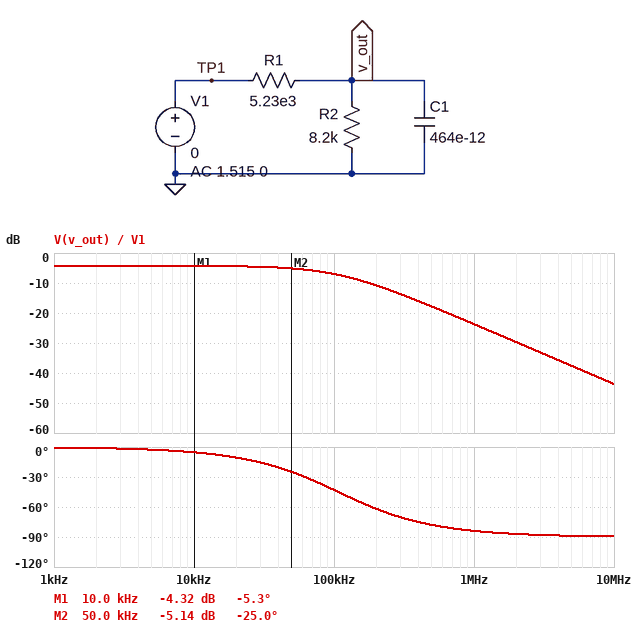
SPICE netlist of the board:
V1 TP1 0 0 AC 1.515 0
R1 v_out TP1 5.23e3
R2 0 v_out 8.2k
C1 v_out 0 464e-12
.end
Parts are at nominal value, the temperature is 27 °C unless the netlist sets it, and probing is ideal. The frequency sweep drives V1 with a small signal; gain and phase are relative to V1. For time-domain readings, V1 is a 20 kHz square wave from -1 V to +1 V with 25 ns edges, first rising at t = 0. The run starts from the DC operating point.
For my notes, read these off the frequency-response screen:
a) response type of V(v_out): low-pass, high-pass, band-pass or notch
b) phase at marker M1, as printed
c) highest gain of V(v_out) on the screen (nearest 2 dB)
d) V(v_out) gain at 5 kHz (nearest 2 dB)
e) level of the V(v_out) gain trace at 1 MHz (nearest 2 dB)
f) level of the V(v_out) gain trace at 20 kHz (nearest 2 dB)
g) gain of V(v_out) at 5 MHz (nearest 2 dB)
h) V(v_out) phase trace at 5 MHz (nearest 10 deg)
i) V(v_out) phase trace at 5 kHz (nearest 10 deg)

low-pass
-5.3 deg
-4 dB
-4 dB
-24 dB
-4 dB
-38 dB
-90 deg
0 deg
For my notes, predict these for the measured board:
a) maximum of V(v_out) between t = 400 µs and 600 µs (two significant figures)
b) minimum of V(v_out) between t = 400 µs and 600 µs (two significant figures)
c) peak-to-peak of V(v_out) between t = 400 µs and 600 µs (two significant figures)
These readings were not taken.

610 mV
-610 mV
1.2 V
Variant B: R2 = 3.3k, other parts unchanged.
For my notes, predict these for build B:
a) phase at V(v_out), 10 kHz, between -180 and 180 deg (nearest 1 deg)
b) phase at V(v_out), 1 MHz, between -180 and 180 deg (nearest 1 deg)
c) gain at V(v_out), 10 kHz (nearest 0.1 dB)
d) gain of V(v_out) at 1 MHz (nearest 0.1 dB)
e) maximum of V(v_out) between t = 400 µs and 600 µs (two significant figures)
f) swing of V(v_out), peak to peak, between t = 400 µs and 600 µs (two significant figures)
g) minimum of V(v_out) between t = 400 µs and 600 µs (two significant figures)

-3 deg
-80 deg
-8.3 dB
-23.8 dB
390 mV
770 mV
-390 mV
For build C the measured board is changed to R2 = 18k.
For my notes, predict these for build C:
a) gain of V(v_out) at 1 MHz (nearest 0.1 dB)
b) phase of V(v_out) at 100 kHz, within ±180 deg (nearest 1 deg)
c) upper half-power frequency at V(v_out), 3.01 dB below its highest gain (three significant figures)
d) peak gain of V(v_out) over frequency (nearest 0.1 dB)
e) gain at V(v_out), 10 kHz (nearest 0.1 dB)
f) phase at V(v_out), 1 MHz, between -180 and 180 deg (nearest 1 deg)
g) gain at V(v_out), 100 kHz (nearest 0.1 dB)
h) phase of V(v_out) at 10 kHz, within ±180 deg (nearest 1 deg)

-23.7 dB
-50 deg
84.6 kHz
-2.2 dB
-2.3 dB
-85 deg
-6.0 dB
-7 deg
